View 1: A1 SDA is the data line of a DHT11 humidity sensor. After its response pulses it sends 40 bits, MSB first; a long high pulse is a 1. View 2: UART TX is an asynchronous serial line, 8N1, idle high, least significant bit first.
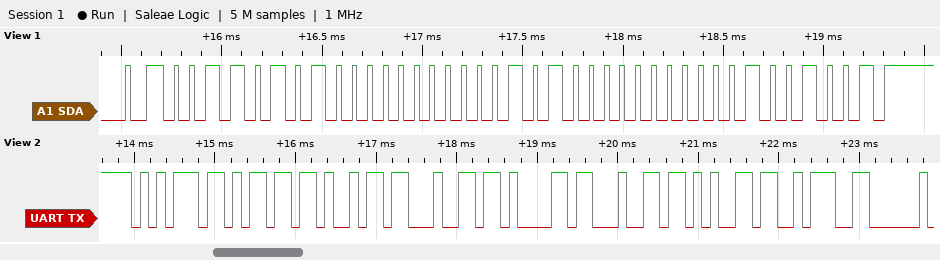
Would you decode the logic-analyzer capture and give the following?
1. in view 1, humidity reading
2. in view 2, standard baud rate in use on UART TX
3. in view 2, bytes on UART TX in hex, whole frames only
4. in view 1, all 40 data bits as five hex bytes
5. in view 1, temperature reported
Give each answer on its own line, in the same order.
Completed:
53 %
9600 baud
75 6D 69 64 61 64 65 3A
35 00 14 00 49
20.0 °C
